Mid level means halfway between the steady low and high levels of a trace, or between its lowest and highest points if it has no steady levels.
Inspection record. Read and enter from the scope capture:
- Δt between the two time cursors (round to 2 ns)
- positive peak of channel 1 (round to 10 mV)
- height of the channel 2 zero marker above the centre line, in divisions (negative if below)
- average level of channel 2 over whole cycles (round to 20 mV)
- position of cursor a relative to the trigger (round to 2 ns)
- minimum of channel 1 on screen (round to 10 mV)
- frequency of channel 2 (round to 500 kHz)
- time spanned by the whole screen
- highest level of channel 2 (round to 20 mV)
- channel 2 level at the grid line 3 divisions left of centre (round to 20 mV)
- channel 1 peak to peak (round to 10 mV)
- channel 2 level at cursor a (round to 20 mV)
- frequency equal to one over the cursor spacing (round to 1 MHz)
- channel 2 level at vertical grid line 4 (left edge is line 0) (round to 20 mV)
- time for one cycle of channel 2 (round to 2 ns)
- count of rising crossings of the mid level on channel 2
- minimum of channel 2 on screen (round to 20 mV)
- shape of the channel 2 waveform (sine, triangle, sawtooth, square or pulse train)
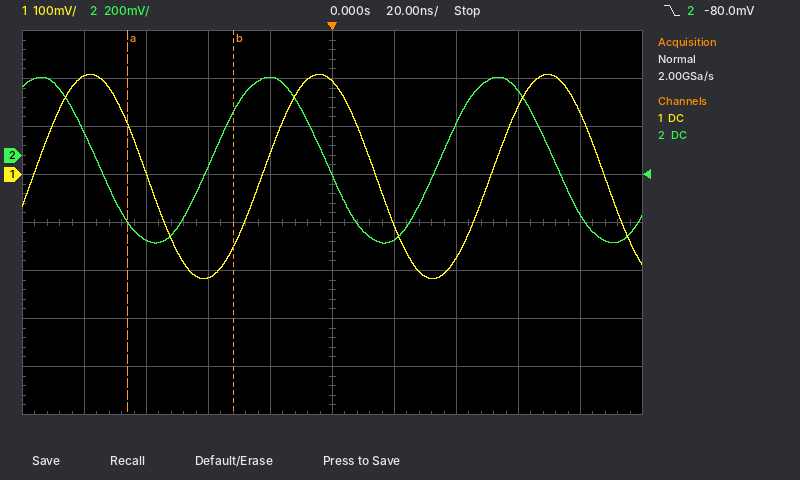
34 ns
210 mV
+1.4 div
-20 mV
-66 ns
-220 mV
13.5 MHz
200 ns
320 mV
-360 mV
430 mV
-280 mV
29 MHz
320 mV
74 ns
2
-360 mV
sine
